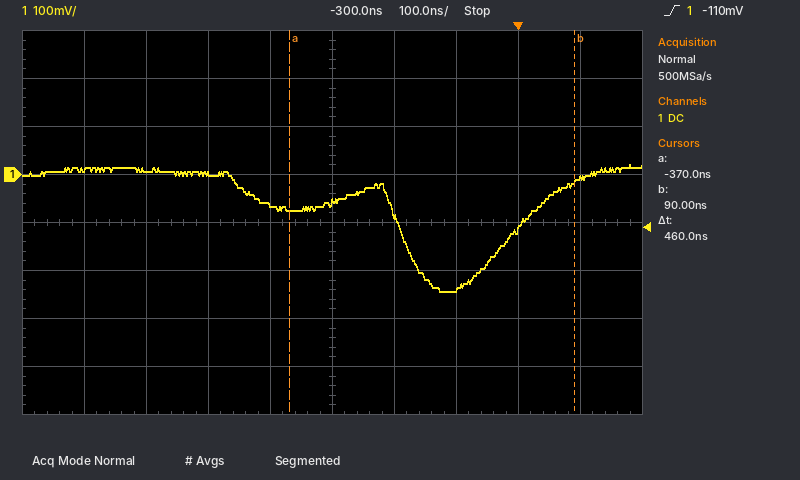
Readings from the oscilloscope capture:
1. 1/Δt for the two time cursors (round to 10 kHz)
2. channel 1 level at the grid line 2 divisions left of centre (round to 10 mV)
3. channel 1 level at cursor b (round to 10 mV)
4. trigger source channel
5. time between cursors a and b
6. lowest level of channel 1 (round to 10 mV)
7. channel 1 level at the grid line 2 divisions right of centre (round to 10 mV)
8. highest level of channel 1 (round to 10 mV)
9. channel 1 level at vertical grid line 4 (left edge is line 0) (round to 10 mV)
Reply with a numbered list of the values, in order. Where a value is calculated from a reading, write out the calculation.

1. 1 / 460 ns ≈ 2.17 MHz
2. 0 mV
3. -20 mV
4. channel 1
5. 460 ns
6. -240 mV
7. -240 mV
8. 20 mV
9. -60 mV
